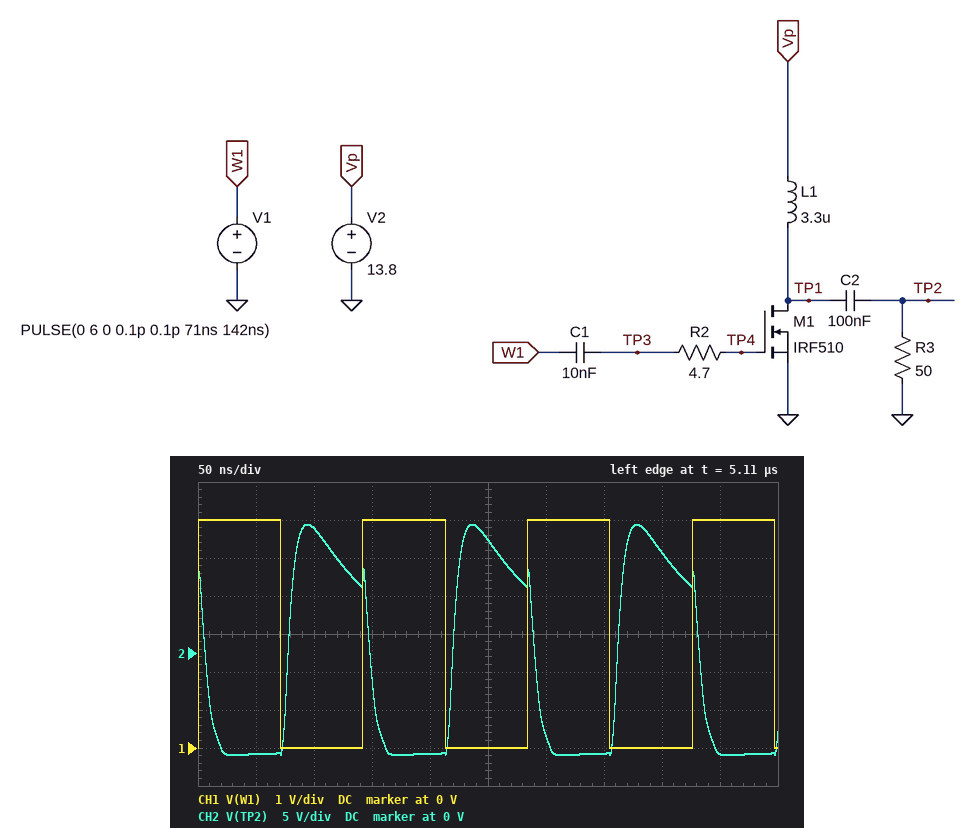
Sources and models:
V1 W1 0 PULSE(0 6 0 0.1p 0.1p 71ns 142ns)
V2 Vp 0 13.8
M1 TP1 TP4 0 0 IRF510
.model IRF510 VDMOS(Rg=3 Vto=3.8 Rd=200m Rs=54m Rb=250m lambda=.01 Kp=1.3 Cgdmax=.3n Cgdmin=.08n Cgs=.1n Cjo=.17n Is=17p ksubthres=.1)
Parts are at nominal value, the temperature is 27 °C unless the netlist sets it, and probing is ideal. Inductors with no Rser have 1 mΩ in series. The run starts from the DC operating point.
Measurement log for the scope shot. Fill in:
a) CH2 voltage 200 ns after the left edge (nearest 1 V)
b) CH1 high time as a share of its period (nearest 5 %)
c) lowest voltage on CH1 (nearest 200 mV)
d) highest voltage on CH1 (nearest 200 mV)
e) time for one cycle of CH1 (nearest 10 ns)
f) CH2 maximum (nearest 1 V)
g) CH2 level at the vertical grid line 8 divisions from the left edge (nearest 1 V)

-13 V
50 %
0 V
6.0 V
140 ns
17 V
13 V
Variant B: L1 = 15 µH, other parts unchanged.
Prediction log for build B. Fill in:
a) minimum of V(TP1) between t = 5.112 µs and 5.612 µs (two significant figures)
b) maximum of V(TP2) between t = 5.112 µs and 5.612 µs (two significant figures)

160 mV
15 V
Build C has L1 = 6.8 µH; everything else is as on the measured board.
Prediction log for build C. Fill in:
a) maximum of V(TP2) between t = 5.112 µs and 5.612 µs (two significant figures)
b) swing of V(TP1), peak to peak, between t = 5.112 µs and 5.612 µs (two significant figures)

15 V
28 V
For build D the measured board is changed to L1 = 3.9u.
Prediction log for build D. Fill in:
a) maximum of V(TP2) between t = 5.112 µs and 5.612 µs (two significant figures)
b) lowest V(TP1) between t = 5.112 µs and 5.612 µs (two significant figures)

16 V
220 mV
